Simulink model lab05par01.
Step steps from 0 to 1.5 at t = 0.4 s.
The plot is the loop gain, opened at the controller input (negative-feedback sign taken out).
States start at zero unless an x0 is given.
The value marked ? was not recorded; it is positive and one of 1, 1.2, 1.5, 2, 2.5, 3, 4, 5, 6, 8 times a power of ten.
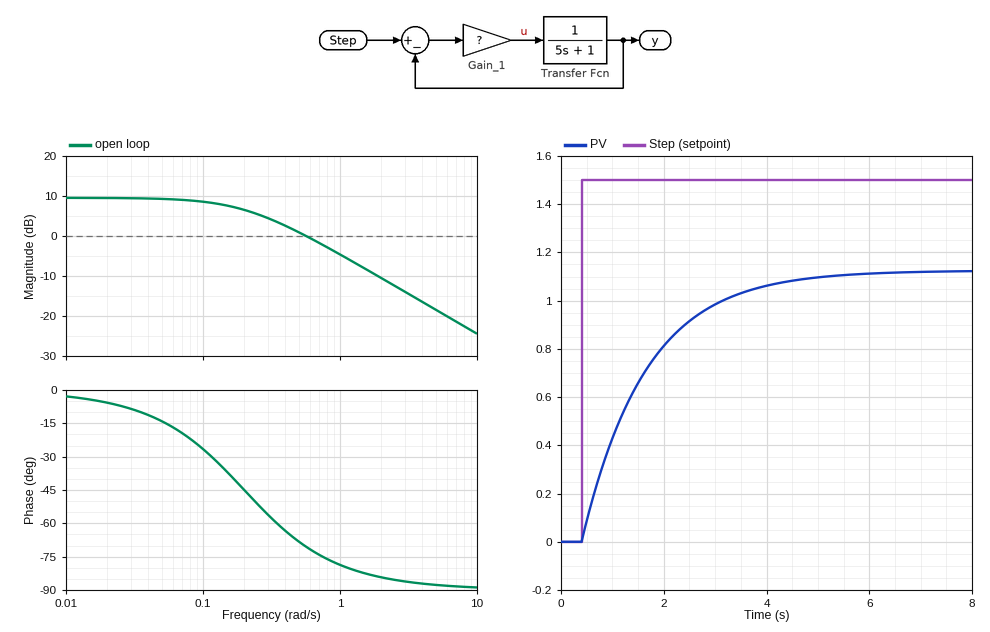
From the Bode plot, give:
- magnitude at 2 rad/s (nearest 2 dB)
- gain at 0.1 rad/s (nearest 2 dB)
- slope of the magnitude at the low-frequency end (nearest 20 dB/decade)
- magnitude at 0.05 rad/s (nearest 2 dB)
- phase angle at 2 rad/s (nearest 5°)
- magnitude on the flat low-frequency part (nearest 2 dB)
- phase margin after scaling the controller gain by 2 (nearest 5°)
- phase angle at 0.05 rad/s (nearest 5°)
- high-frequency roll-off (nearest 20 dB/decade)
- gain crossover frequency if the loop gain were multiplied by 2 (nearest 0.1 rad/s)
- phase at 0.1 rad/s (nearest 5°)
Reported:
-10 dB
8 dB
0 dB/decade
10 dB
-85°
10 dB
100°
-15°
-20 dB/decade
1.2 rad/s
-25°
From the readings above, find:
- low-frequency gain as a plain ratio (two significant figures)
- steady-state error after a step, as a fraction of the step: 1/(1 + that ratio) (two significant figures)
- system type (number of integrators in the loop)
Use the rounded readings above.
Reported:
3.2
0.24
0
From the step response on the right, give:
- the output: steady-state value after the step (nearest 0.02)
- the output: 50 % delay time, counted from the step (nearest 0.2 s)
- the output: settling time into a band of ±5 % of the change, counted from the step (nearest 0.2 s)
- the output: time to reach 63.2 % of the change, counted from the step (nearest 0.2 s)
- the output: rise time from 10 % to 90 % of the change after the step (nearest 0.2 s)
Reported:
1.12
0.8 s
3.8 s
1.2 s
2.8 s
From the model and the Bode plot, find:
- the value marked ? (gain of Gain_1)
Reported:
3
